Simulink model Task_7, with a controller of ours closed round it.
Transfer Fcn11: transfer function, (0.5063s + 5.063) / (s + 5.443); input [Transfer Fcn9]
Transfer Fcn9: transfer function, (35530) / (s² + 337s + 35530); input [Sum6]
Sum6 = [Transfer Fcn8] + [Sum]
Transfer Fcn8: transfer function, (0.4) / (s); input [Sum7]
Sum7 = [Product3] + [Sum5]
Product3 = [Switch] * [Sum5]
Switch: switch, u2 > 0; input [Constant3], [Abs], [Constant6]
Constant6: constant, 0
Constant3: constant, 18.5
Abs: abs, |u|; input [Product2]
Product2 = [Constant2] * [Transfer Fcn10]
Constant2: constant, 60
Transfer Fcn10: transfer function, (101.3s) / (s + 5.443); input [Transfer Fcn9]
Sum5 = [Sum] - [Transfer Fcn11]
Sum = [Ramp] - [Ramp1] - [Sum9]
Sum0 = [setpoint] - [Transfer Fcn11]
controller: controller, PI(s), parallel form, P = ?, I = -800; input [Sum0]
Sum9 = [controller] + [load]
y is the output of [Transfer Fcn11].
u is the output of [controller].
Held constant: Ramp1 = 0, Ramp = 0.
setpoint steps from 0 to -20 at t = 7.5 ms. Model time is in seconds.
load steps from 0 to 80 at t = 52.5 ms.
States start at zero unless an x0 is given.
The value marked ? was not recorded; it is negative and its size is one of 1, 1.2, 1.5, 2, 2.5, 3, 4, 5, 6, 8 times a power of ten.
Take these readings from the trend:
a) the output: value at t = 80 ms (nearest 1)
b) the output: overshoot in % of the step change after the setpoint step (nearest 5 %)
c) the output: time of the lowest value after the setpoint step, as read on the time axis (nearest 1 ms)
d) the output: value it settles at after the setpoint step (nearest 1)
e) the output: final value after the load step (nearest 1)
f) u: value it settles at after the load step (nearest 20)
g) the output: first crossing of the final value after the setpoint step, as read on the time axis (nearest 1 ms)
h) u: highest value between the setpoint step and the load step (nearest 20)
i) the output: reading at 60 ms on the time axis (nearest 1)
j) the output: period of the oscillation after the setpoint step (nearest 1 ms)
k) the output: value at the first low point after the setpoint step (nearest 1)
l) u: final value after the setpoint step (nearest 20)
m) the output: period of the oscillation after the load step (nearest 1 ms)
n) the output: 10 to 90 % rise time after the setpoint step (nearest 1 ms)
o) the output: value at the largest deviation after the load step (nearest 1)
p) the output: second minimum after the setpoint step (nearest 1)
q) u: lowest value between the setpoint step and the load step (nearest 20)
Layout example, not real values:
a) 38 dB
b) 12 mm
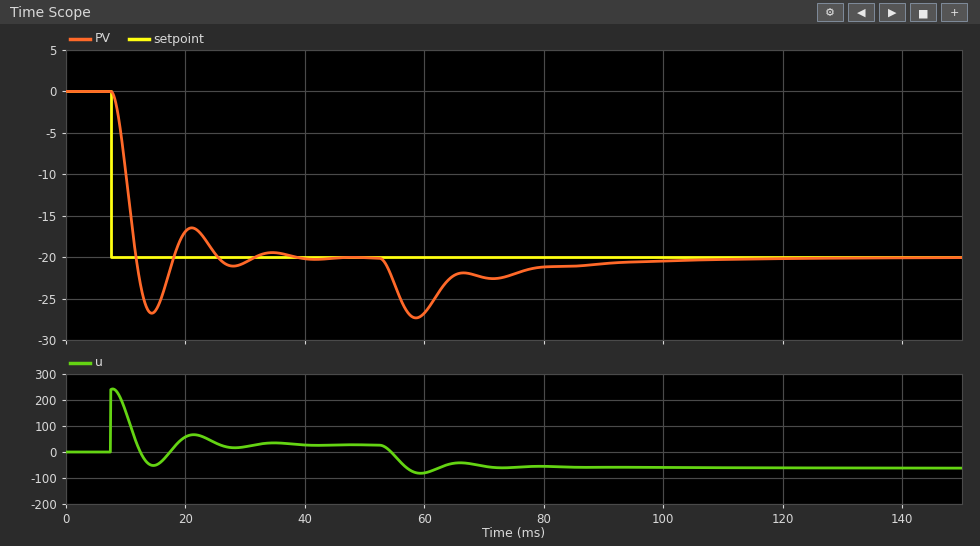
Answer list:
a) -21
b) 35 %
c) 14 ms
d) -20
e) -20
f) -60
g) 12 ms
h) 240
i) -27
j) 14 ms
k) -27
l) 20
m) 13 ms
n) 3 ms
o) -27
p) -21
q) -60
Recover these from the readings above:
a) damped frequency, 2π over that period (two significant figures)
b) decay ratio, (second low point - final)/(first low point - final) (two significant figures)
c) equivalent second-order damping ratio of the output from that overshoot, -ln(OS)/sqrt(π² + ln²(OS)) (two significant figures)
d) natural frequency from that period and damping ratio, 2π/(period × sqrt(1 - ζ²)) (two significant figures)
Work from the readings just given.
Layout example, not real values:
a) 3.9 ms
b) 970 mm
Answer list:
a) 0.45 rad/ms
b) 0.14
c) 0.32
d) 0.47 rad/ms
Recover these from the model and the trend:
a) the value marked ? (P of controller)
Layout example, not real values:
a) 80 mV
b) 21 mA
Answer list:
a) -12
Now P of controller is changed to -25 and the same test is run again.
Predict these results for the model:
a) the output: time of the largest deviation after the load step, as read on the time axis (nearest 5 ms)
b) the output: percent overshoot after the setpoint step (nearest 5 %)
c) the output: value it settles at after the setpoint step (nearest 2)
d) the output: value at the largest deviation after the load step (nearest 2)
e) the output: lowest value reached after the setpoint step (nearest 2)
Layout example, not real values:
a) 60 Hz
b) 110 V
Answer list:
a) 55 ms
b) 45 %
c) -20
d) -24
e) -28
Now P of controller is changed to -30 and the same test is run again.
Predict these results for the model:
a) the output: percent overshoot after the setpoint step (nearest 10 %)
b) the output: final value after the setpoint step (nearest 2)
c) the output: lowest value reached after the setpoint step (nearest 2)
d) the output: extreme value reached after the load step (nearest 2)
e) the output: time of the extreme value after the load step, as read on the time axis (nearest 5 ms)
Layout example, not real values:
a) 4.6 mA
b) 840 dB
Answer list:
a) 50 %
b) -20
c) -30
d) -24
e) 55 ms
